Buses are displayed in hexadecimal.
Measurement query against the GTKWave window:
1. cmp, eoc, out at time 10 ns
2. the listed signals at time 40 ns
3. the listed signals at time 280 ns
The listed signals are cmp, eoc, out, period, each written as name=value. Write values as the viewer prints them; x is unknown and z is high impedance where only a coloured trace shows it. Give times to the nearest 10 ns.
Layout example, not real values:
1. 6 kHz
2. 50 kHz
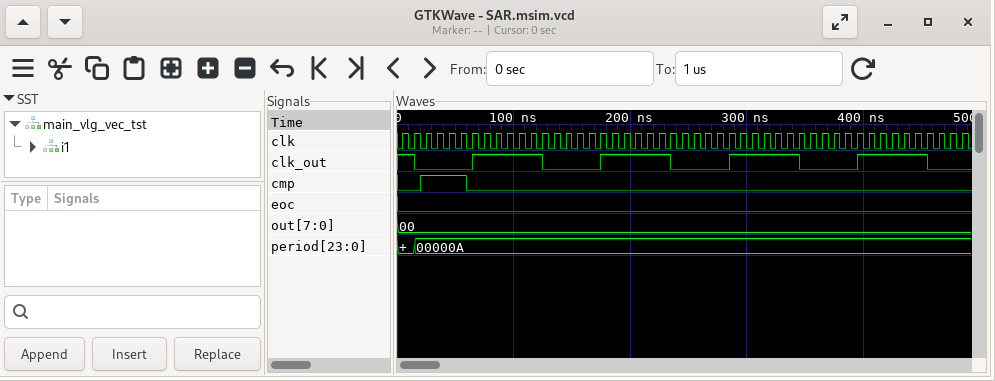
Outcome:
1. cmp=0, eoc=0, out=00
2. cmp=1, eoc=0, out=00, period=00000A
3. cmp=0, eoc=0, out=00, period=00000A
